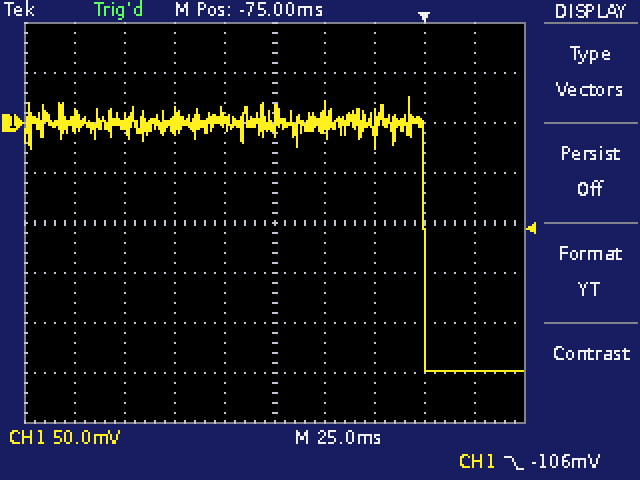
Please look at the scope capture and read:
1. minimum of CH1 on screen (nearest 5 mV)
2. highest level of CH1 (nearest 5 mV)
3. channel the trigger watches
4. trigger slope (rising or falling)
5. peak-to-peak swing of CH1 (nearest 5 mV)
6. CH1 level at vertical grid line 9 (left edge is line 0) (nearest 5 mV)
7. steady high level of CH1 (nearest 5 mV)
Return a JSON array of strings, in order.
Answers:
["-250 mV", "25 mV", "CH1", "falling", "275 mV", "-250 mV", "0 mV"]
